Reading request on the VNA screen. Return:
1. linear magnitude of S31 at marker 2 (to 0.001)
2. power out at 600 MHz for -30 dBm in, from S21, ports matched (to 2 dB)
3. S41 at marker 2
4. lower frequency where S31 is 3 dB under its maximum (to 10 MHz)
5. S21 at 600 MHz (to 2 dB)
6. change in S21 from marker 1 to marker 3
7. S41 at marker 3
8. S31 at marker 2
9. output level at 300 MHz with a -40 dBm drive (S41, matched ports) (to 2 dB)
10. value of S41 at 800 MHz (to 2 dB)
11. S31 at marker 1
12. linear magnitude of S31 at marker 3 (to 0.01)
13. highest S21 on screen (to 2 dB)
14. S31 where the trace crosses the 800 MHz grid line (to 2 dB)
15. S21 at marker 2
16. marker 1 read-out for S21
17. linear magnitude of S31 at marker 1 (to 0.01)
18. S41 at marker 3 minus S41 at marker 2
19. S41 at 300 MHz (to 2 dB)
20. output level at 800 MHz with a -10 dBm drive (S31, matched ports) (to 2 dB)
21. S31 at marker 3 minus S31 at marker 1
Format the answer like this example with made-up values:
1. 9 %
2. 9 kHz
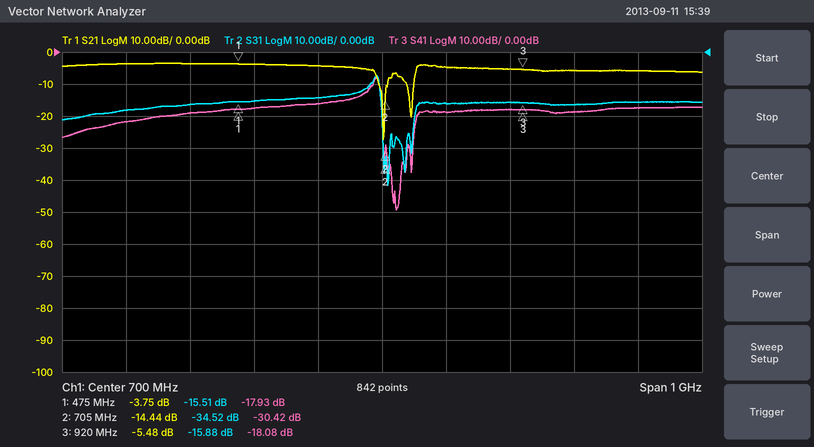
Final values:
1. 0.019
2. -34 dBm
3. -30.42 dB
4. 680 MHz
5. -4 dB
6. -1.73 dB
7. -18.08 dB
8. -34.52 dB
9. -62 dBm
10. -18 dB
11. -15.51 dB
12. 0.16
13. -4 dB
14. -16 dB
15. -14.44 dB
16. -3.75 dB
17. 0.17
18. 12.34 dB
19. -22 dB
20. -26 dBm
21. -0.37 dB
